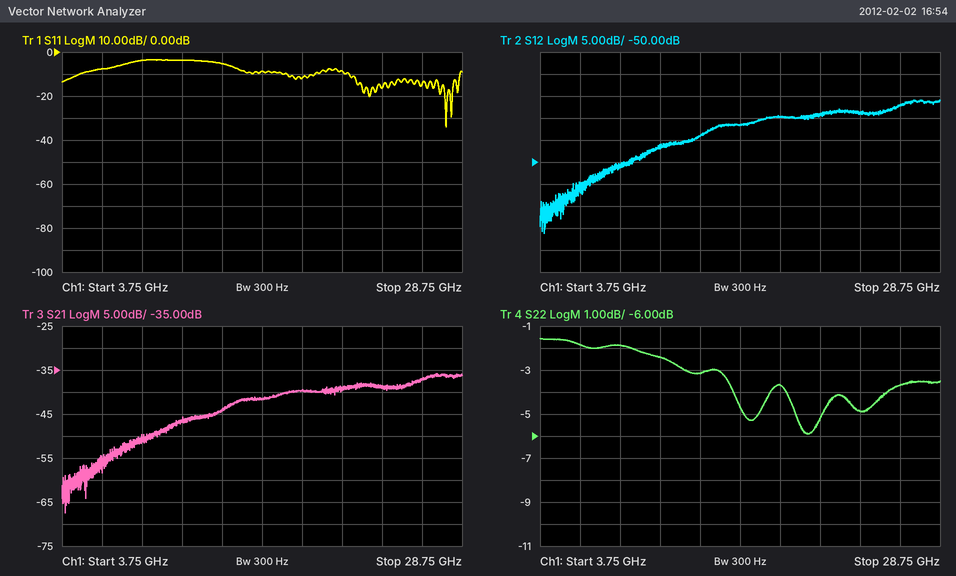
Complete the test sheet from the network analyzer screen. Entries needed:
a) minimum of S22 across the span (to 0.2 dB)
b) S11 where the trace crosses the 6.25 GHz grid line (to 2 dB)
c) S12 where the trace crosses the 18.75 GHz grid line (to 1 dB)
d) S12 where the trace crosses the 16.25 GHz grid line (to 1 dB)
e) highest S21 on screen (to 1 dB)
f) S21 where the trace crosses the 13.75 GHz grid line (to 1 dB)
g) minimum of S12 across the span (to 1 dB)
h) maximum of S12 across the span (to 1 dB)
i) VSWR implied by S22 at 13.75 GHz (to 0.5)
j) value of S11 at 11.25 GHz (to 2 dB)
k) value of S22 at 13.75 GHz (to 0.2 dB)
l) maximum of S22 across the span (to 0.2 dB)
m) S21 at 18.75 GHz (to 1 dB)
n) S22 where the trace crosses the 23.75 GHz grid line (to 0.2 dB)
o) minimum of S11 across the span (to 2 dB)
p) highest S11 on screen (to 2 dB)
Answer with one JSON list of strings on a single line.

["-6.0 dB", "-8 dB", "-40 dB", "-42 dB", "-36 dB", "-44 dB", "-66 dB", "-36 dB", "5.5", "-4 dB", "-3.2 dB", "-1.6 dB", "-40 dB", "-4.8 dB", "-34 dB", "-4 dB"]
